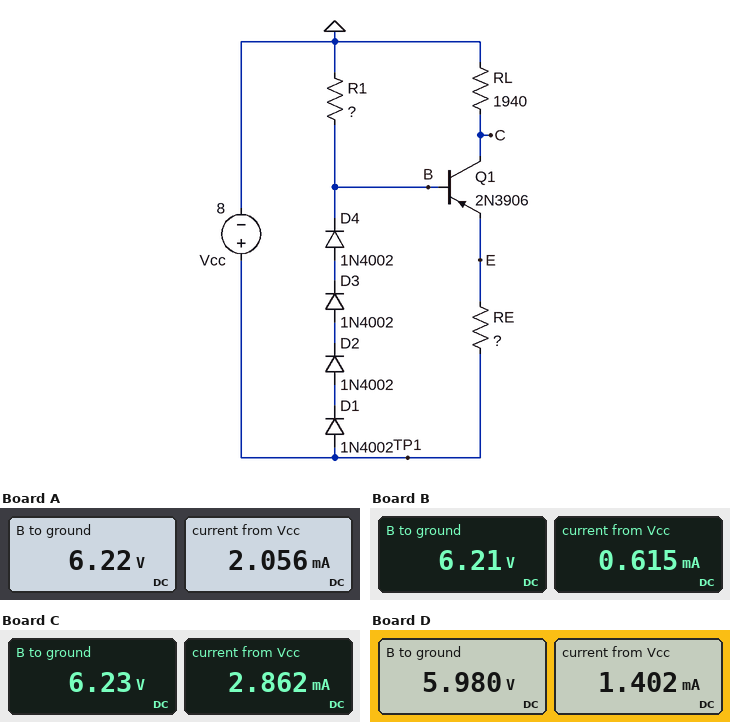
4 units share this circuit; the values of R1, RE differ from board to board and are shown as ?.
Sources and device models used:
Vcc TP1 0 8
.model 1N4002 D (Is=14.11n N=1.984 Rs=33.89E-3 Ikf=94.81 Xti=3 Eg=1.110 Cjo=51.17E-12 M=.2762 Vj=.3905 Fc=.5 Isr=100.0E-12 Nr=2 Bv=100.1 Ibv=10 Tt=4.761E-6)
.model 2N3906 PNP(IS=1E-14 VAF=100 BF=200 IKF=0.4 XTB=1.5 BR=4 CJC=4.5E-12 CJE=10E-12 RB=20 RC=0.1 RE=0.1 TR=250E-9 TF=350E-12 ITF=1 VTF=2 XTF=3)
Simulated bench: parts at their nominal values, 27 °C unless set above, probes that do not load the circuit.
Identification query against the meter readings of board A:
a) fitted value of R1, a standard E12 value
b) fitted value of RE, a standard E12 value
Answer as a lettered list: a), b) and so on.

a) 68 kΩ
b) 560 Ω
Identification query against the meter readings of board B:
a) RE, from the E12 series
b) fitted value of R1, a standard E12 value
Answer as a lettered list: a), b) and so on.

a) 2.2 kΩ
b) 68 kΩ
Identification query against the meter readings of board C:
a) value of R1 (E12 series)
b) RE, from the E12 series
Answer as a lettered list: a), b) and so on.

a) 68 kΩ
b) 390 Ω
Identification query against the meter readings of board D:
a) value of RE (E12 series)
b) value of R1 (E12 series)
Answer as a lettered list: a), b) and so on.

a) 1.2 kΩ
b) 22 kΩ
